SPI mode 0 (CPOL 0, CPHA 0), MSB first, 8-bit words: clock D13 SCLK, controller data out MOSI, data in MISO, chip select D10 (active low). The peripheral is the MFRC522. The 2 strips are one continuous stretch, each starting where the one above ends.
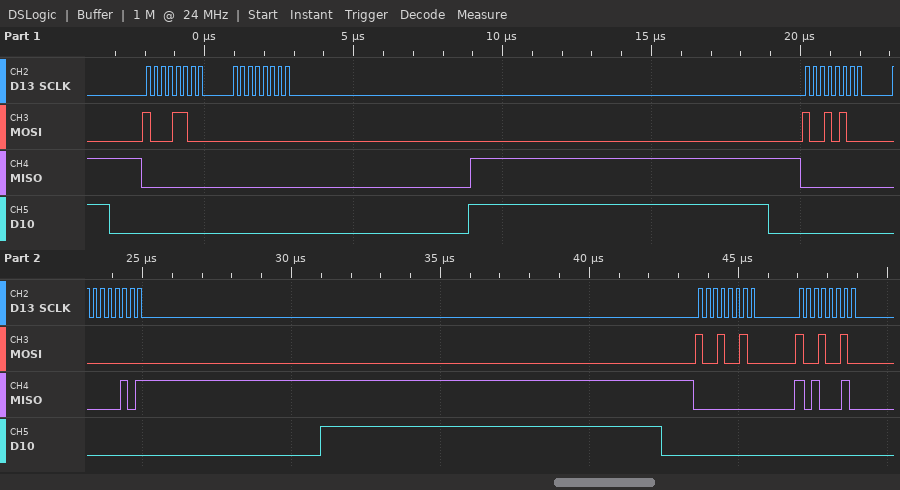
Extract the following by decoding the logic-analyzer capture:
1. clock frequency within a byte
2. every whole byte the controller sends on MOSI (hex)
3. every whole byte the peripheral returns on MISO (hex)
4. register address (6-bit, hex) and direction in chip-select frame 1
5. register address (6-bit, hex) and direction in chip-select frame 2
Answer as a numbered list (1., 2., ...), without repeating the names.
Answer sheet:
1. 4 MHz
2. 0x8C 0x00 0x94 0x00 0x92 0x92
3. 0x00 0x00 0x00 0x05 0x00 0xA2
4. 0x06 read
5. 0x0A read
